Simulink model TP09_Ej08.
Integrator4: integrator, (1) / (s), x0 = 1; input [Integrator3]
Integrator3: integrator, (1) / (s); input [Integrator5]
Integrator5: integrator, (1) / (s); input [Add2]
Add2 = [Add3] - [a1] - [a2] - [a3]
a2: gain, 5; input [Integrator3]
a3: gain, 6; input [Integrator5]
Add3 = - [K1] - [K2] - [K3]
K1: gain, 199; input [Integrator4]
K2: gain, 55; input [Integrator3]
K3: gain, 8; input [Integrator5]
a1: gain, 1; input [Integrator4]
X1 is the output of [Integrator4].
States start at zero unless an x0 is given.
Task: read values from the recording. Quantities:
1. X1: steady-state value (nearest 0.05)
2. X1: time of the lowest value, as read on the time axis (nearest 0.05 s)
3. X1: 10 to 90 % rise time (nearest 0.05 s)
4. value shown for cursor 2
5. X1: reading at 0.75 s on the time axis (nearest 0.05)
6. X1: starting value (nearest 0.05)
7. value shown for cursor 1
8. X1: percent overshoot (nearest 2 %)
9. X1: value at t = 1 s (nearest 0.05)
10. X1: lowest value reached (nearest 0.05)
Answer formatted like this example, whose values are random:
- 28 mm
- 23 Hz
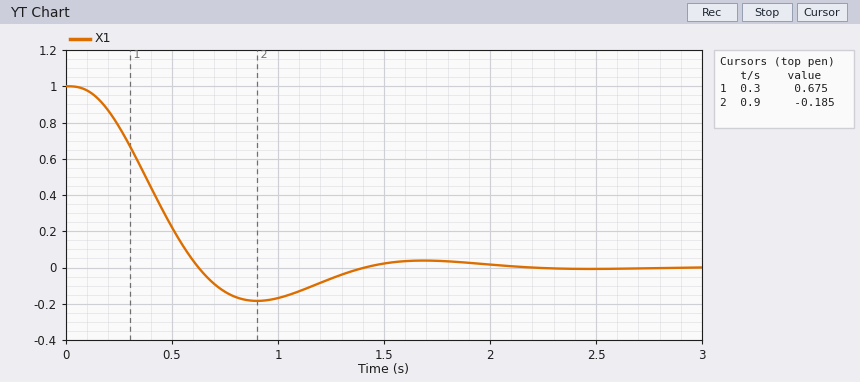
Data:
- 0.00
- 0.90 s
- 0.40 s
- -0.185
- -0.15
- 1.00
- 0.675
- 18 %
- -0.15
- -0.20
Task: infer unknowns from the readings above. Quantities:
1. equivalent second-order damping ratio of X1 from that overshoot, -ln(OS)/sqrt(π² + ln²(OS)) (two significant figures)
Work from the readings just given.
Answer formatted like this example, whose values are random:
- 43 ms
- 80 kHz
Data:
- 0.48
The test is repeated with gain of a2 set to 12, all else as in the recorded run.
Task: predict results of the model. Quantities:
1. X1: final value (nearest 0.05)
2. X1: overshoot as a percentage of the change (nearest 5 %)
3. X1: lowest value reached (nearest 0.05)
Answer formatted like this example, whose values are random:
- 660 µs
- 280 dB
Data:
- 0.00
- 10 %
- -0.10
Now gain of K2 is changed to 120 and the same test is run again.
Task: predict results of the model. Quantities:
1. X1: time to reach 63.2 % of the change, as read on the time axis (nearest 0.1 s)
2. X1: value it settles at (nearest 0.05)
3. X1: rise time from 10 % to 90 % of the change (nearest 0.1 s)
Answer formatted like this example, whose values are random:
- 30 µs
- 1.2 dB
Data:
- 0.6 s
- 0.00
- 1.1 s
